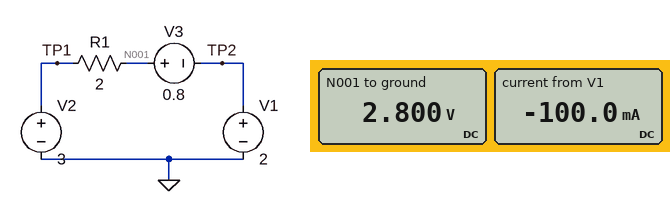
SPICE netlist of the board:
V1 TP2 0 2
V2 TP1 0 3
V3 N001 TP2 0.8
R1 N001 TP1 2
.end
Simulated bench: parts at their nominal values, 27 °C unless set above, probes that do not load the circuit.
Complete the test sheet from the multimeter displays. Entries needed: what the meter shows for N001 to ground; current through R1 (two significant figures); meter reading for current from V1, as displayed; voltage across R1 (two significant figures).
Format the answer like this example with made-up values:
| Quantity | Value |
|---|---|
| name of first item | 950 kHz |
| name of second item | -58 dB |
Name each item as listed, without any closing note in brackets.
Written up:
| Quantity | Value |
|---|---|
| what the meter shows for N001 to ground | 2.800 V |
| current through R1 | 100 mA |
| meter reading for current from V1, as displayed | -100.0 mA |
| voltage across R1 | 200 mV |
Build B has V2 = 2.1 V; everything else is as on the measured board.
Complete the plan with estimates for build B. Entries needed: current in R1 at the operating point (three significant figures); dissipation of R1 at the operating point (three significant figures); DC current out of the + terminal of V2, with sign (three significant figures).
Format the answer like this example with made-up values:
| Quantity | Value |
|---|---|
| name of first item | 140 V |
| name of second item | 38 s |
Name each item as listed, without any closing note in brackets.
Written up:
| Quantity | Value |
|---|---|
| current in R1 at the operating point | 350 mA |
| dissipation of R1 at the operating point | 245 mW |
| DC current out of the + terminal of V2, with sign | -350 mA |
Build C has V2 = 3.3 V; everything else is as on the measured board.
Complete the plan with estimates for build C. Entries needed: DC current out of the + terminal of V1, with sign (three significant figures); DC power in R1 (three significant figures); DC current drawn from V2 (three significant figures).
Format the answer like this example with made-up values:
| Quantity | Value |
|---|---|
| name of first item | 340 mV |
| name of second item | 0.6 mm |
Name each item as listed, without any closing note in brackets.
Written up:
| Quantity | Value |
|---|---|
| DC current out of the + terminal of V1, with sign | -250 mA |
| DC power in R1 | 125 mW |
| DC current drawn from V2 | 250 mA |
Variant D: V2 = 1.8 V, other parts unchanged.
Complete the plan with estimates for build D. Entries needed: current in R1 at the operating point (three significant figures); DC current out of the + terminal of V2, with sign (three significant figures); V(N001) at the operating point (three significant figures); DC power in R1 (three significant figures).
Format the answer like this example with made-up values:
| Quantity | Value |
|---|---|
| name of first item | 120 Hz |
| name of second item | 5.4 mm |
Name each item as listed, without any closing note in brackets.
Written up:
| Quantity | Value |
|---|---|
| current in R1 at the operating point | 500 mA |
| DC current out of the + terminal of V2, with sign | -500 mA |
| V(N001) at the operating point | 2.80 V |
| DC power in R1 | 500 mW |
